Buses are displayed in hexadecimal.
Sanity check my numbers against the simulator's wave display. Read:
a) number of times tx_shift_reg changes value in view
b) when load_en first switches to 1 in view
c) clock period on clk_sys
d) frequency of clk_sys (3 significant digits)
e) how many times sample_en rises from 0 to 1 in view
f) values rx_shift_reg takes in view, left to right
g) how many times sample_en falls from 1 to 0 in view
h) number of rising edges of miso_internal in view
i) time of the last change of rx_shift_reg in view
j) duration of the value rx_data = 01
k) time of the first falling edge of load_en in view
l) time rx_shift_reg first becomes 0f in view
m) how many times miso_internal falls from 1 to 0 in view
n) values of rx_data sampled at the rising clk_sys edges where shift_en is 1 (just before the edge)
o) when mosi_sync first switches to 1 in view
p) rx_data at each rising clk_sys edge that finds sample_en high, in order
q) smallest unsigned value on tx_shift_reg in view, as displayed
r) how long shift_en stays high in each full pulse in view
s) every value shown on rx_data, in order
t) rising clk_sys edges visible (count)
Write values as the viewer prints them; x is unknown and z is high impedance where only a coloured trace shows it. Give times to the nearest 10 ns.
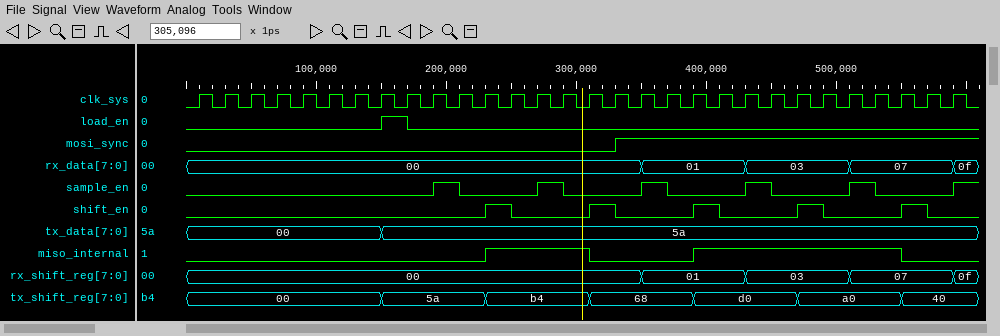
6
150 ns
20 ns
50.0 MHz
6
00, 01, 03, 07, 0f
5
2
590 ns
80 ns
170 ns
590 ns
2
00, 00, 01, 03, 07
330 ns
00, 00, 01, 03, 07
00
20 ns, 20 ns, 20 ns, 20 ns, 20 ns
00, 01, 03, 07, 0f
30
